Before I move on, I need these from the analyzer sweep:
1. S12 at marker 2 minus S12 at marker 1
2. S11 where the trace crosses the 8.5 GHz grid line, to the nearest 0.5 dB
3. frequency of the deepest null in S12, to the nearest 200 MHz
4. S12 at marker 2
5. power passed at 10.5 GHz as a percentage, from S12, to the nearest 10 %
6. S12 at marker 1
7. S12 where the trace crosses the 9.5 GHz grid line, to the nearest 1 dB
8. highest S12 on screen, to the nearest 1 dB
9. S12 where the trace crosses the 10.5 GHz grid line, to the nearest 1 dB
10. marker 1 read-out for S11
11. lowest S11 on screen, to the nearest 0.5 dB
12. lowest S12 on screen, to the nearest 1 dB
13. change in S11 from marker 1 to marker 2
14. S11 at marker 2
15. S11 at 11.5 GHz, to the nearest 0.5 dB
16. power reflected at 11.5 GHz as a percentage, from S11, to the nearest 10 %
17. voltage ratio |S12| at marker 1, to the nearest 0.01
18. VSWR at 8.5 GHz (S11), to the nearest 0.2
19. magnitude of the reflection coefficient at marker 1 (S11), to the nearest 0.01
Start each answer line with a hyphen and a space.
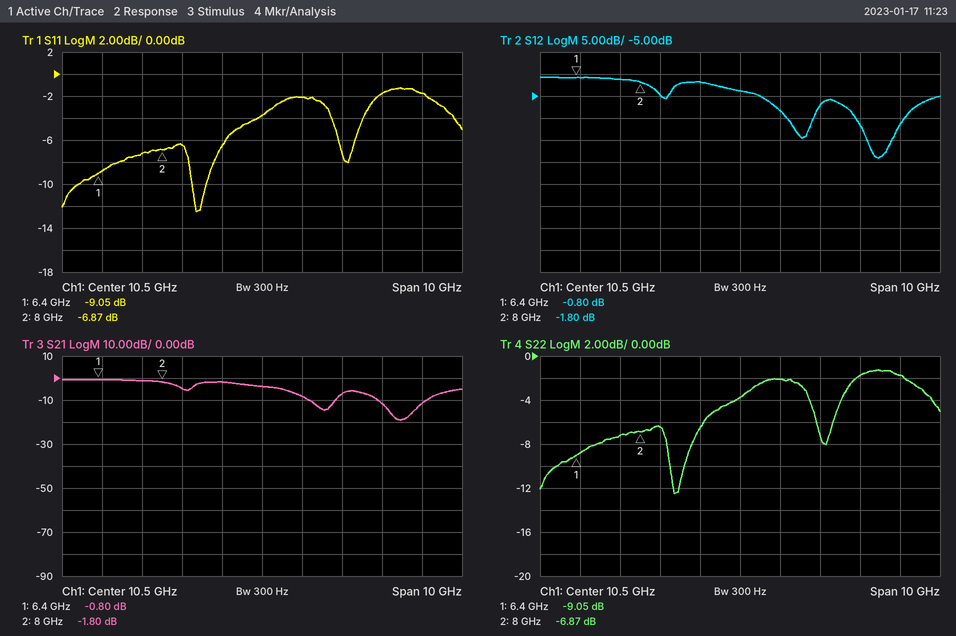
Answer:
- -1.00 dB
- -6.5 dB
- 14.0 GHz
- -1.80 dB
- 40 %
- -0.80 dB
- -2 dB
- -1 dB
- -4 dB
- -9.05 dB
- -12.5 dB
- -19 dB
- 2.18 dB
- -6.87 dB
- -2.0 dB
- 60 %
- 0.91
- 2.8
- 0.35
